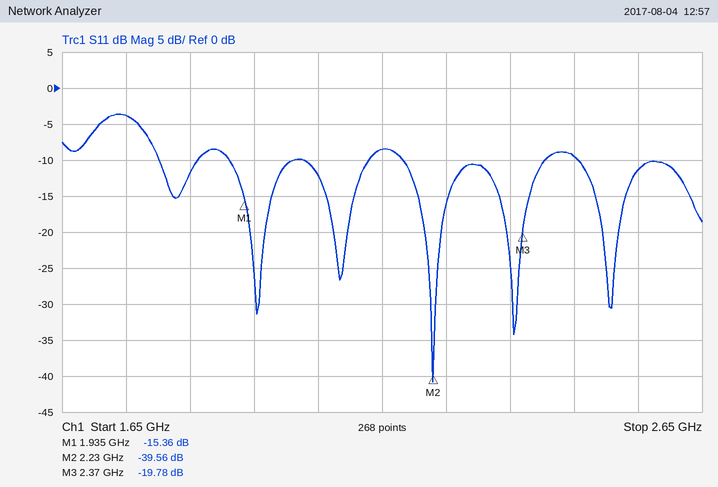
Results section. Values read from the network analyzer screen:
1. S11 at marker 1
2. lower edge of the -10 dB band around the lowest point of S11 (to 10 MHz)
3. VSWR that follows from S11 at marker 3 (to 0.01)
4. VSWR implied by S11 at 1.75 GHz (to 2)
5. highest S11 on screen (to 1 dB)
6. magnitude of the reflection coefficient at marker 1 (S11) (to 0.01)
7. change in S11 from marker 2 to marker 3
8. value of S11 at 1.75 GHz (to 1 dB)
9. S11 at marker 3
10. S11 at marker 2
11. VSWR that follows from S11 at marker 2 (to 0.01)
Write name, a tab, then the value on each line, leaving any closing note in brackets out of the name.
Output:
S11 at marker 1	-15.36 dB
lower edge of the -10 dB band around the lowest point of S11	2.18 GHz
VSWR that follows from S11 at marker 3	1.23
VSWR implied by S11 at 1.75 GHz	4
highest S11 on screen	-4 dB
magnitude of the reflection coefficient at marker 1 (S11)	0.17
change in S11 from marker 2 to marker 3	19.78 dB
value of S11 at 1.75 GHz	-4 dB
S11 at marker 3	-19.78 dB
S11 at marker 2	-39.56 dB
VSWR that follows from S11 at marker 2	1.02
